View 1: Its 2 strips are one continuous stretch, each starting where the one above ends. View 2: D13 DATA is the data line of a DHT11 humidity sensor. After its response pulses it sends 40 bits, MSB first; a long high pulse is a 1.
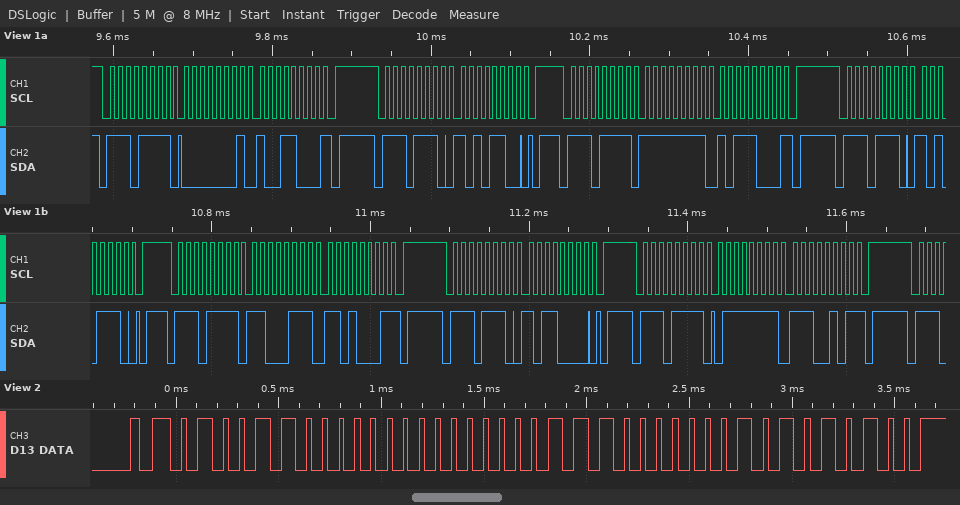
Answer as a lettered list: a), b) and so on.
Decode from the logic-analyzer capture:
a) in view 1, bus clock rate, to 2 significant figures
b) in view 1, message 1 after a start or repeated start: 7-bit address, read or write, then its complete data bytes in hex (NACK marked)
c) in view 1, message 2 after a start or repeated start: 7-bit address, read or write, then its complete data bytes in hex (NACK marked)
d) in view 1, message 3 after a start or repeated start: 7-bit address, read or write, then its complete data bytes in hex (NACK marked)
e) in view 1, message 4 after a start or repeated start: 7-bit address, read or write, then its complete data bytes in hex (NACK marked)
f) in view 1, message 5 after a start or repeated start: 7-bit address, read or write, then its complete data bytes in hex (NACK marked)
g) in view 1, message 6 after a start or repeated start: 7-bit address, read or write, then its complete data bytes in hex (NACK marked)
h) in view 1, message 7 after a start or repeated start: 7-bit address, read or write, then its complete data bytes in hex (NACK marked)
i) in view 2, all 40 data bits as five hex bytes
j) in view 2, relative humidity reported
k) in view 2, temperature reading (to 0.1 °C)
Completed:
a) 100 kHz
b) 0x77 read: 01 98 NACK
c) 0x77 write: AC
d) 0x77 read: FF B8 NACK
e) 0x77 write: AE
f) 0x77 read: C7 D1 NACK
g) 0x77 write: B0
h) 0x77 read: 7F E5 NACK
i) 4C 00 07 01 54
j) 76 %
k) 7.1 °C
